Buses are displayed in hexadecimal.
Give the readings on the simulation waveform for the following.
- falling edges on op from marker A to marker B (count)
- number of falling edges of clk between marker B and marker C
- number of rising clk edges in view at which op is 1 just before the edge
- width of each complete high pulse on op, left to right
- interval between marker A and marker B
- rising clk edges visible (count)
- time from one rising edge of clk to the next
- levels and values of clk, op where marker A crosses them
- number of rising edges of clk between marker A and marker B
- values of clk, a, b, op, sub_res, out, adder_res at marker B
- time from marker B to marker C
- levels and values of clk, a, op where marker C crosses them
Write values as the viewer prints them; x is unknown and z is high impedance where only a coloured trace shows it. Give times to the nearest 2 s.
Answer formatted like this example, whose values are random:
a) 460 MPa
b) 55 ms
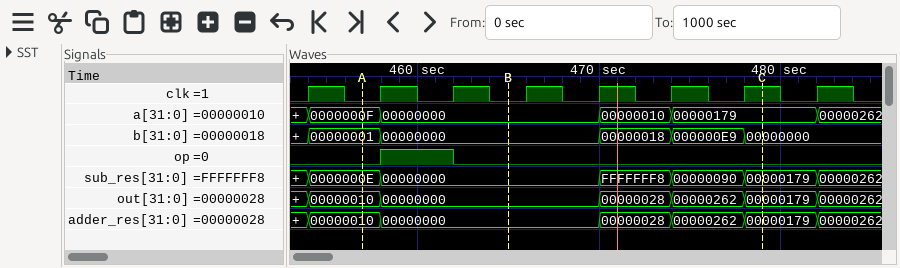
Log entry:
a) 1
b) 3
c) 1
d) 4 s
e) 8 s
f) 8
g) 4 s
h) clk=0, op=0
i) 2
j) clk=0, a=00000000, b=00000000, op=0, sub_res=00000000, out=00000000, adder_res=00000000
k) 14 s
l) clk=1, a=00000179, op=0
